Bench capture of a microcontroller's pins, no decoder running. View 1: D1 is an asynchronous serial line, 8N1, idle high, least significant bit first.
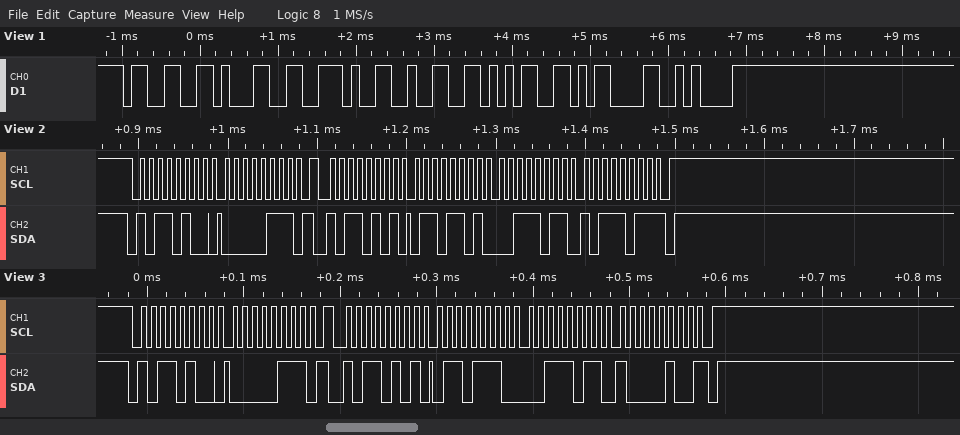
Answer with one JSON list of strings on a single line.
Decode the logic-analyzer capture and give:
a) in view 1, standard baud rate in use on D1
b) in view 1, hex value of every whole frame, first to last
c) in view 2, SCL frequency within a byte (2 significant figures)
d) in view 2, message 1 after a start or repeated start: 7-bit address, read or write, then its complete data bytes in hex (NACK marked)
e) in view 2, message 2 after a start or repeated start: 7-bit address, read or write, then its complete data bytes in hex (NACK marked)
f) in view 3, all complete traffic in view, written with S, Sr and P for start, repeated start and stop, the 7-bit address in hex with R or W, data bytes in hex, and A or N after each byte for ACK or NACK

["9600 baud", "0x33 0x31 0x2E 0x32 0x35 0x0D 0x0A", "100 kHz", "0x5A write: 07", "0x5A read: 6D 3B BB NACK", "S 5AW A 07 A Sr 5AR A 6E A 3B A 84 N P"]
